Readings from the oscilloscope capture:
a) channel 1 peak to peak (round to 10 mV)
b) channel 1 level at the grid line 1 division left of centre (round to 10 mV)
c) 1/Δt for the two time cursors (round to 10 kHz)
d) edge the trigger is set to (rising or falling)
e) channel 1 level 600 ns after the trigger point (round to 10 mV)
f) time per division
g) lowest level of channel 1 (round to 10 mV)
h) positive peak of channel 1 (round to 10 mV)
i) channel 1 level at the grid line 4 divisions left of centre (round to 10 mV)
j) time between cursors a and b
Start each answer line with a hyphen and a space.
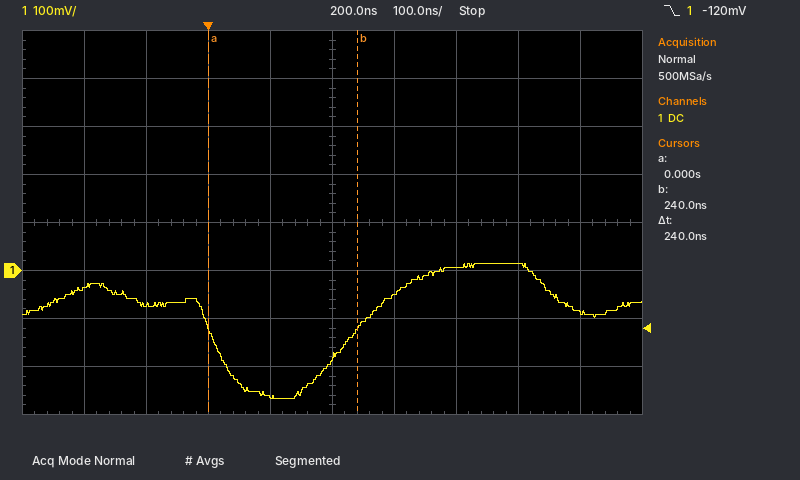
- 280 mV
- -260 mV
- 4.17 MHz
- falling
- -90 mV
- 100 ns
- -270 mV
- 10 mV
- -40 mV
- 240 ns
